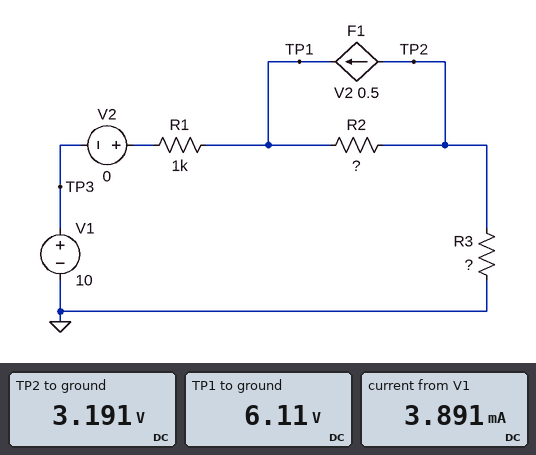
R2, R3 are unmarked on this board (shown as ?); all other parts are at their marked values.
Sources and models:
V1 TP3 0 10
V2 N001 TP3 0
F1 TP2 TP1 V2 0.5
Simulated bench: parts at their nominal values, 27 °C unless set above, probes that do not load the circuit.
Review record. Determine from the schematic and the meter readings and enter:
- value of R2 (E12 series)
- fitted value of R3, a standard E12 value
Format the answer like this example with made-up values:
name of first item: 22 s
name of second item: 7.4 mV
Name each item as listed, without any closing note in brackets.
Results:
value of R2: 1.5 kΩ
fitted value of R3, a standard E12 value: 820 Ω
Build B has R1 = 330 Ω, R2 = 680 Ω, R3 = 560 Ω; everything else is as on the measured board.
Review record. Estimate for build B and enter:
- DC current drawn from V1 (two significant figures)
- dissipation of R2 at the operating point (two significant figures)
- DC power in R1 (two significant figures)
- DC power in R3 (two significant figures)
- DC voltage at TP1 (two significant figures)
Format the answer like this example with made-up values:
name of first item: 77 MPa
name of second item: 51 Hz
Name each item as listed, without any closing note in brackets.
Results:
DC current drawn from V1: 8.1 mA
dissipation of R2 at the operating point: 11 mW
DC power in R1: 22 mW
DC power in R3: 37 mW
DC voltage at TP1: 7.3 V
